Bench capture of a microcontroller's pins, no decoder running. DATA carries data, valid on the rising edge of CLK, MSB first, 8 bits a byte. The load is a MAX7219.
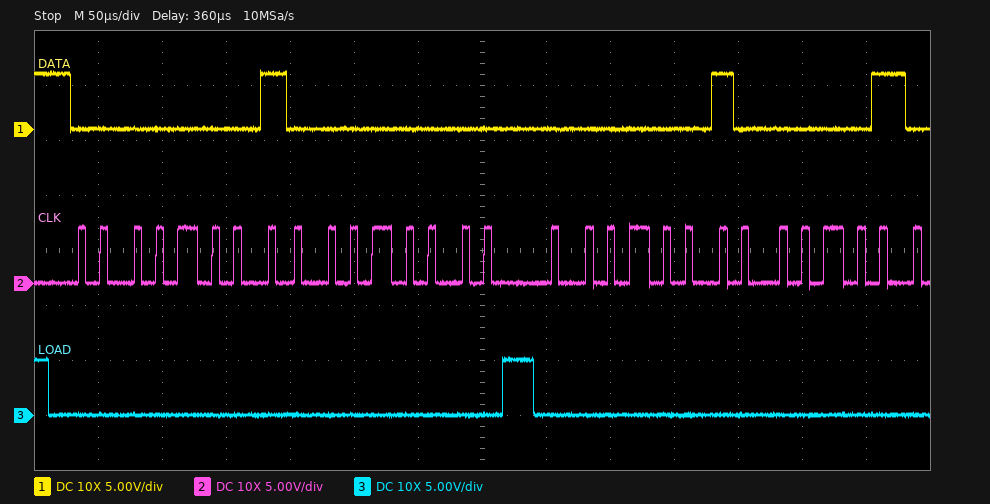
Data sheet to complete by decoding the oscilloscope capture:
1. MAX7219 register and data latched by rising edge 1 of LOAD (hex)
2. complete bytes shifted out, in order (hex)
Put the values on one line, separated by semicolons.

register 0x1, data 0x00; 01 00 02
